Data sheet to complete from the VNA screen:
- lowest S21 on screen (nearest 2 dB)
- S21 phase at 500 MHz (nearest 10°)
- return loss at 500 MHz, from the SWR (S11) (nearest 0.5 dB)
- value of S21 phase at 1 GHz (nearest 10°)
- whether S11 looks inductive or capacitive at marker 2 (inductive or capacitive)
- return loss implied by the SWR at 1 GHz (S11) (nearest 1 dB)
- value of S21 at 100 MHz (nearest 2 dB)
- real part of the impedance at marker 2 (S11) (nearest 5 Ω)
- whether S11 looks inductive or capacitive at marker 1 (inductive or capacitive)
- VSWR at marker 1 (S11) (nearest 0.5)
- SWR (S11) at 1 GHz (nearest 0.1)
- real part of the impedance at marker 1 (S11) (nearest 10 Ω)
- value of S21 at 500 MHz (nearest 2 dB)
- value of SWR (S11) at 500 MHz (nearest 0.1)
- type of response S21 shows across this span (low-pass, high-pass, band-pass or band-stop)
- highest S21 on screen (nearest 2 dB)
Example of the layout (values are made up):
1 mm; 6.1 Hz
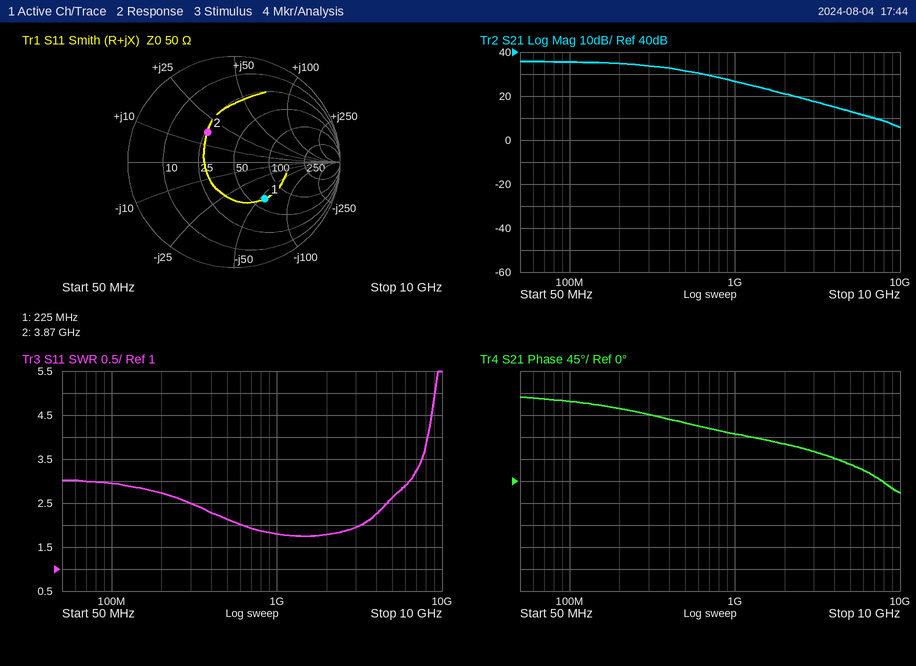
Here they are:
6 dB; 120°; 9.0 dB; 100°; inductive; 11 dB; 36 dB; 25 Ω; capacitive; 2.5; 1.8; 60 Ω; 32 dB; 2.1; low-pass; 36 dB
